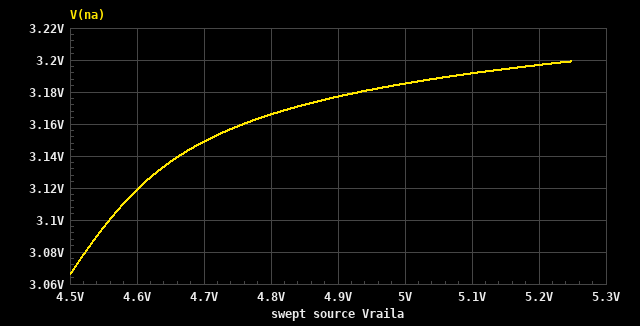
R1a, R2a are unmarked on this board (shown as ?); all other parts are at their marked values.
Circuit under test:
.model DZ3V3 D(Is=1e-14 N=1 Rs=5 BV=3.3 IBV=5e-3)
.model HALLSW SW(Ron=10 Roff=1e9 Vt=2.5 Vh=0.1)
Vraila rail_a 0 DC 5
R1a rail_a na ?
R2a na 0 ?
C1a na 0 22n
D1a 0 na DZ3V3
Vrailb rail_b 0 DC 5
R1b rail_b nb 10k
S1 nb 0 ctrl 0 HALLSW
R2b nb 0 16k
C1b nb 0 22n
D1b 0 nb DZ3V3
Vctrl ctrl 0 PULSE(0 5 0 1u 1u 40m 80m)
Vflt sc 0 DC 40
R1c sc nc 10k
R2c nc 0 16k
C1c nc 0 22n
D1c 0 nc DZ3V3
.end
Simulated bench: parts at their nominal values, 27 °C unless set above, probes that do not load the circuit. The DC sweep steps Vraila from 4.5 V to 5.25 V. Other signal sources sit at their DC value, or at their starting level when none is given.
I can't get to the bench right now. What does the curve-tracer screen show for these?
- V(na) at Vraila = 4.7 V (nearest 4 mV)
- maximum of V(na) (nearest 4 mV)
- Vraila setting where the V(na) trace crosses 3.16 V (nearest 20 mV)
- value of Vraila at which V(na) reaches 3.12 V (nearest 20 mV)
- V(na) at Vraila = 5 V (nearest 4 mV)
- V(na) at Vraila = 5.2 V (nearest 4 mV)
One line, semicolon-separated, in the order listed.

3.148 V; 3.200 V; 4.76 V; 4.60 V; 3.184 V; 3.196 V
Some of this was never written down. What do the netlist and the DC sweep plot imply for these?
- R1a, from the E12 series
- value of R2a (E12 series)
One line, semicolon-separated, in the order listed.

5.6 kΩ; 12 kΩ
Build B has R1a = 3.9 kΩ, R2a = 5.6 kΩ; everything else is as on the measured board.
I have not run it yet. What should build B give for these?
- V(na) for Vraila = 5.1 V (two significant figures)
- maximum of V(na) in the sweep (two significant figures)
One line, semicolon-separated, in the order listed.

3.0 V; 3.1 V
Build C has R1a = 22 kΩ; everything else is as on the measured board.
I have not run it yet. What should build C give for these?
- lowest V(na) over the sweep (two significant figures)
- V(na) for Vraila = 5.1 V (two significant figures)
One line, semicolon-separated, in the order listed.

1.6 V; 1.8 V
